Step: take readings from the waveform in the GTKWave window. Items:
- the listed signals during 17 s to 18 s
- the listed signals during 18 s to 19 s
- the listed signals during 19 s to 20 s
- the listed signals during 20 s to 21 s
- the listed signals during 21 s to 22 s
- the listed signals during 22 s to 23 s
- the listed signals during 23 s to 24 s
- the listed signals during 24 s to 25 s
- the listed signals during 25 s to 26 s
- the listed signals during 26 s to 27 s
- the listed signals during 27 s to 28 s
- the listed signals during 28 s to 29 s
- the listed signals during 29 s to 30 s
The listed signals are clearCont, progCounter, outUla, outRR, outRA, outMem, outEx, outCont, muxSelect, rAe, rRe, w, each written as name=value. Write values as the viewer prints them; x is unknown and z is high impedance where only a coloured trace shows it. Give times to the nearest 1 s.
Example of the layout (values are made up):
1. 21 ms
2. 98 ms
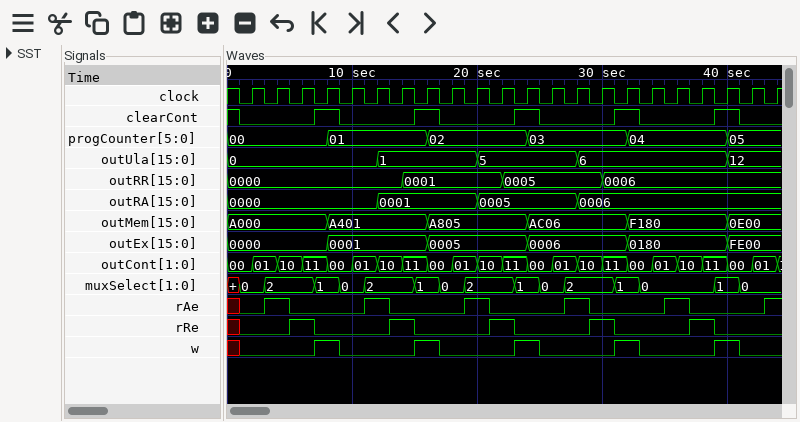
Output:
1. clearCont=0, progCounter=02, outUla=1, outRR=0001, outRA=0001, outMem=A805, outEx=0005, outCont=00, muxSelect=0, rAe=0, rRe=0, w=0
2. clearCont=0, progCounter=02, outUla=1, outRR=0001, outRA=0001, outMem=A805, outEx=0005, outCont=01, muxSelect=0, rAe=0, rRe=0, w=0
3. clearCont=0, progCounter=02, outUla=1, outRR=0001, outRA=0001, outMem=A805, outEx=0005, outCont=01, muxSelect=2, rAe=1, rRe=0, w=0
4. clearCont=0, progCounter=02, outUla=5, outRR=0001, outRA=0005, outMem=A805, outEx=0005, outCont=10, muxSelect=2, rAe=1, rRe=0, w=0
5. clearCont=0, progCounter=02, outUla=5, outRR=0001, outRA=0005, outMem=A805, outEx=0005, outCont=10, muxSelect=2, rAe=0, rRe=1, w=0
6. clearCont=0, progCounter=02, outUla=5, outRR=0005, outRA=0005, outMem=A805, outEx=0005, outCont=11, muxSelect=2, rAe=0, rRe=1, w=0
7. clearCont=1, progCounter=02, outUla=5, outRR=0005, outRA=0005, outMem=A805, outEx=0005, outCont=11, muxSelect=1, rAe=0, rRe=0, w=1
8. clearCont=1, progCounter=03, outUla=5, outRR=0005, outRA=0005, outMem=AC06, outEx=0006, outCont=00, muxSelect=1, rAe=0, rRe=0, w=1
9. clearCont=0, progCounter=03, outUla=5, outRR=0005, outRA=0005, outMem=AC06, outEx=0006, outCont=00, muxSelect=0, rAe=0, rRe=0, w=0
10. clearCont=0, progCounter=03, outUla=5, outRR=0005, outRA=0005, outMem=AC06, outEx=0006, outCont=01, muxSelect=0, rAe=0, rRe=0, w=0
11. clearCont=0, progCounter=03, outUla=5, outRR=0005, outRA=0005, outMem=AC06, outEx=0006, outCont=01, muxSelect=2, rAe=1, rRe=0, w=0
12. clearCont=0, progCounter=03, outUla=6, outRR=0005, outRA=0006, outMem=AC06, outEx=0006, outCont=10, muxSelect=2, rAe=1, rRe=0, w=0
13. clearCont=0, progCounter=03, outUla=6, outRR=0005, outRA=0006, outMem=AC06, outEx=0006, outCont=10, muxSelect=2, rAe=0, rRe=1, w=0
